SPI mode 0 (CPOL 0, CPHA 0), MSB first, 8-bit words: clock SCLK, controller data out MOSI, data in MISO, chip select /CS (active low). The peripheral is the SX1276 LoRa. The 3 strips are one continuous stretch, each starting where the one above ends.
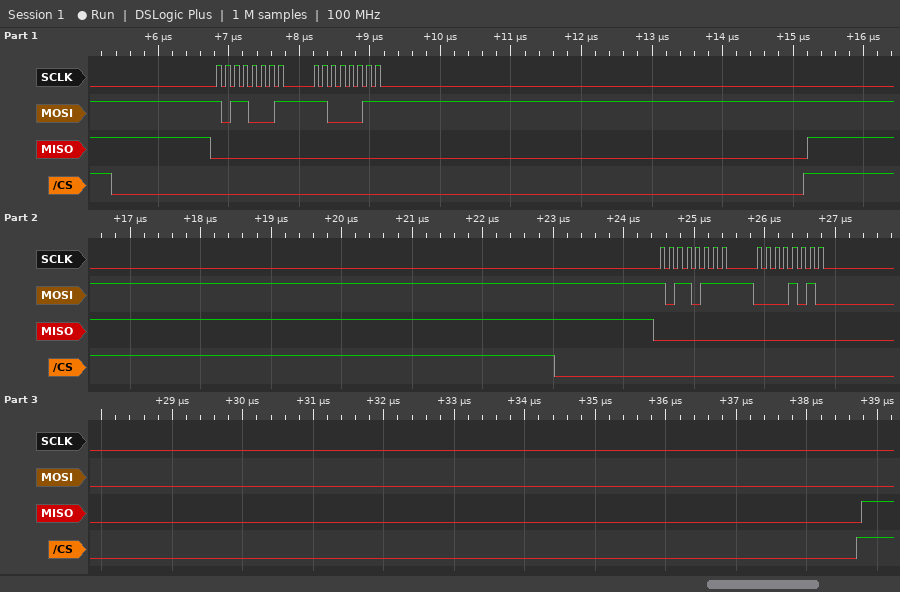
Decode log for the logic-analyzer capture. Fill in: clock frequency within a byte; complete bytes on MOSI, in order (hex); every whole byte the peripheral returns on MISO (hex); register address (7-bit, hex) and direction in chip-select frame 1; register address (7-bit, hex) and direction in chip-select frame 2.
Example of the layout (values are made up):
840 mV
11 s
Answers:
8 MHz
0xB1 0xC3 0xB7 0x0A
0x00 0x00 0x00 0x00
0x31 write
0x37 write
